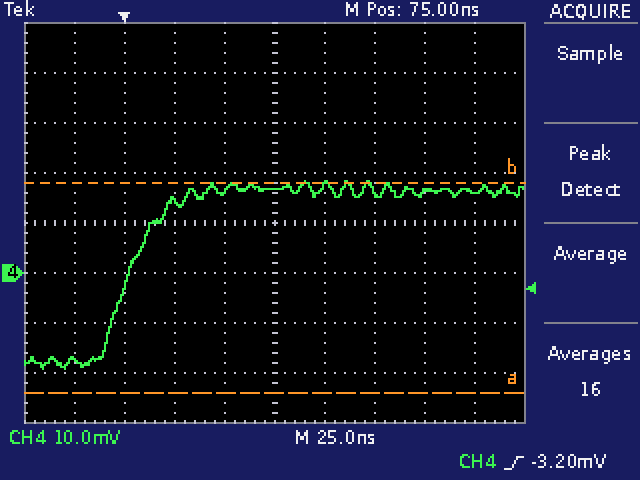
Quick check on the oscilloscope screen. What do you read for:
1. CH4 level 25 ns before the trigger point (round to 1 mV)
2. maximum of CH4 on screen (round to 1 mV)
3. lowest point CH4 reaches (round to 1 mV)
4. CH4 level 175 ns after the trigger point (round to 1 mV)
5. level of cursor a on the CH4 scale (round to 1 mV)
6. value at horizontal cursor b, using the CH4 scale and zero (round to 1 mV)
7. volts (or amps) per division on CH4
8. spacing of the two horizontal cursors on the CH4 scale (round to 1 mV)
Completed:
-17 mV
18 mV
-19 mV
16 mV
-24 mV
18 mV
10 mV
42 mV
